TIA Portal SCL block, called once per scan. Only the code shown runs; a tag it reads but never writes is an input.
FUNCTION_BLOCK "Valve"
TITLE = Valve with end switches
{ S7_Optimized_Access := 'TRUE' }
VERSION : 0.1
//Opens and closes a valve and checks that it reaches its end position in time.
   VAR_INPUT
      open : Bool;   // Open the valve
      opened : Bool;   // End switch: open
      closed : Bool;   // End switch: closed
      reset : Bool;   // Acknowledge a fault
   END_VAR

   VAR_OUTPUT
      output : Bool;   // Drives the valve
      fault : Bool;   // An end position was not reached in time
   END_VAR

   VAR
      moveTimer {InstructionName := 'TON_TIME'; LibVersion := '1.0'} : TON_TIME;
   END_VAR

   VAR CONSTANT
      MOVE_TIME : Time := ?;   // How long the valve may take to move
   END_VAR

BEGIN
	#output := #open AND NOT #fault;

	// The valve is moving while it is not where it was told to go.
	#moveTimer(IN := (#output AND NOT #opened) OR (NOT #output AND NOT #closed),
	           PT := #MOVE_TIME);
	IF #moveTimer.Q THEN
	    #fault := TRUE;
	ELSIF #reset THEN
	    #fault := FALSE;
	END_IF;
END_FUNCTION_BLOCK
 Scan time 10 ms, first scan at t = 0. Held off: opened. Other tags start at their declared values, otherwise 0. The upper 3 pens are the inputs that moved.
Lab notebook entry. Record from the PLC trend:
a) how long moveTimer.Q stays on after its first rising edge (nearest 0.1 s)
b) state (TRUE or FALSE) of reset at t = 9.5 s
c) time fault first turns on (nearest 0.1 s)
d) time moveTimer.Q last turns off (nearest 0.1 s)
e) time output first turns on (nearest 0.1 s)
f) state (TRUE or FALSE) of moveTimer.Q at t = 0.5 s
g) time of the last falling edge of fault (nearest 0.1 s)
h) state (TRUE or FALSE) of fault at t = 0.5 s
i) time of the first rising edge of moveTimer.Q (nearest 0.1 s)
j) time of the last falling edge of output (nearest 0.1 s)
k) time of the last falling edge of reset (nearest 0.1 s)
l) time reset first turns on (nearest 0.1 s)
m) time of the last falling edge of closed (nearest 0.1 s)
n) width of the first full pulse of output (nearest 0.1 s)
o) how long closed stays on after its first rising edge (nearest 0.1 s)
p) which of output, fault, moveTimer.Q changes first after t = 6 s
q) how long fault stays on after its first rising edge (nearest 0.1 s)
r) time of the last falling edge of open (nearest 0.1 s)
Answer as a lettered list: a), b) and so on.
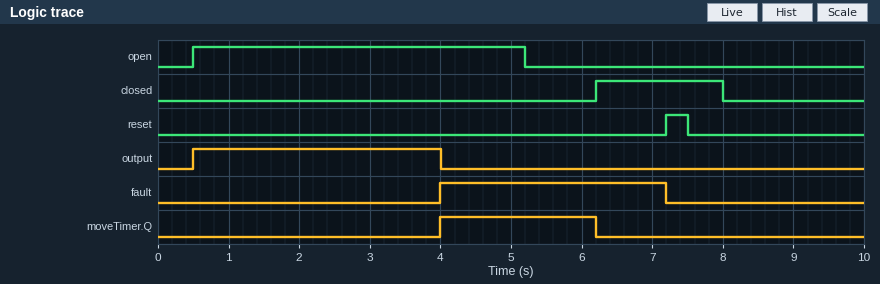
a) 2.2 s
b) FALSE
c) 4.0 s
d) 6.2 s
e) 0.5 s
f) FALSE
g) 7.2 s
h) FALSE
i) 4.0 s
j) 4.0 s
k) 7.5 s
l) 7.2 s
m) 8.0 s
n) 3.5 s
o) 1.8 s
p) moveTimer.Q
q) 3.2 s
r) 5.2 s
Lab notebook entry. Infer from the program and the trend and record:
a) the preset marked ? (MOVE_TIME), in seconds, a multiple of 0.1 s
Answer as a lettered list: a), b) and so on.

a) 4.0 s
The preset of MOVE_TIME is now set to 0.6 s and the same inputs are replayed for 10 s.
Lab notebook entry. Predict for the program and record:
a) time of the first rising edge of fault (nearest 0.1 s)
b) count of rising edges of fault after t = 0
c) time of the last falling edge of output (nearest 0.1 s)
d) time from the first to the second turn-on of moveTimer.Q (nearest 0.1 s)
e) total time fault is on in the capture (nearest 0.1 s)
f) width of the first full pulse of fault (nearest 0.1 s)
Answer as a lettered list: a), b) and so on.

a) 0.6 s
b) 2
c) 0.6 s
d) 8.0 s
e) 8.0 s
f) 6.6 s
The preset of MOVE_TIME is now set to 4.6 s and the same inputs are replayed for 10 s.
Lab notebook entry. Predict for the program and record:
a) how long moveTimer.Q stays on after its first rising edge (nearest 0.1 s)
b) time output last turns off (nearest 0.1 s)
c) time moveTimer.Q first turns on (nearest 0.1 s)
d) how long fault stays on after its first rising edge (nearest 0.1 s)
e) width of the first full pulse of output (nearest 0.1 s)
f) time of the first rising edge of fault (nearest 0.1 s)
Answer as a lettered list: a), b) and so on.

a) 1.6 s
b) 4.6 s
c) 4.6 s
d) 2.6 s
e) 4.1 s
f) 4.6 s
